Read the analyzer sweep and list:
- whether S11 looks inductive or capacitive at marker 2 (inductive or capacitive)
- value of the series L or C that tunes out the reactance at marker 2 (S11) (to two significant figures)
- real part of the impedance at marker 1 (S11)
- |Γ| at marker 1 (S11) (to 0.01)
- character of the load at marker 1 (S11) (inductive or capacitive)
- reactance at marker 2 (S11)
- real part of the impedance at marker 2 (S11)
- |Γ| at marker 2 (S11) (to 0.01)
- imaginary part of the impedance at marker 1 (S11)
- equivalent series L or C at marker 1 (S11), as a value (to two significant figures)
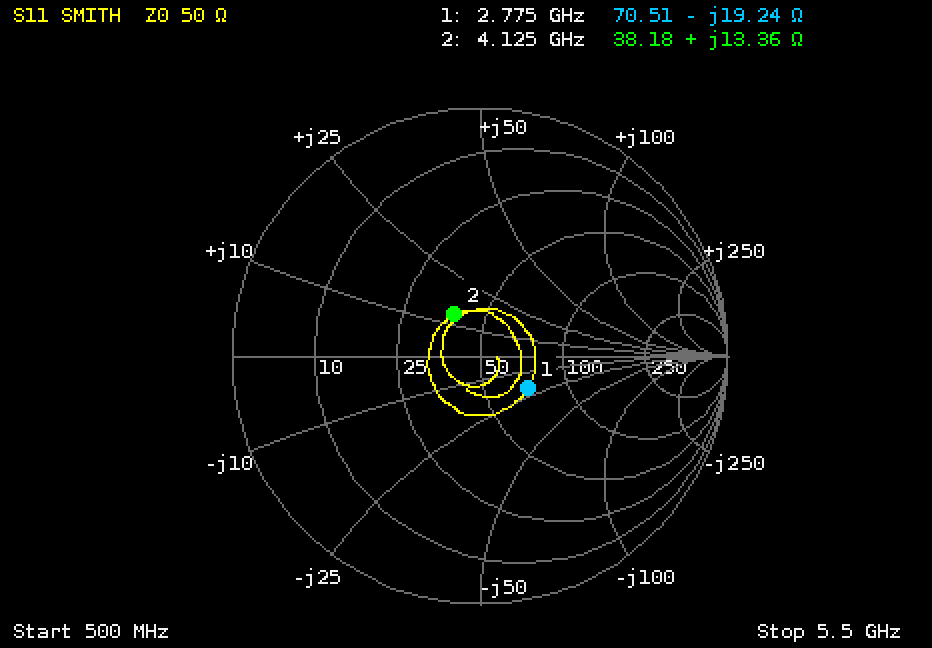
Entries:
inductive
2.9 pF
70.51 Ω
0.23
capacitive
+13.36 Ω
38.18 Ω
0.20
-19.24 Ω
3.0 pF
